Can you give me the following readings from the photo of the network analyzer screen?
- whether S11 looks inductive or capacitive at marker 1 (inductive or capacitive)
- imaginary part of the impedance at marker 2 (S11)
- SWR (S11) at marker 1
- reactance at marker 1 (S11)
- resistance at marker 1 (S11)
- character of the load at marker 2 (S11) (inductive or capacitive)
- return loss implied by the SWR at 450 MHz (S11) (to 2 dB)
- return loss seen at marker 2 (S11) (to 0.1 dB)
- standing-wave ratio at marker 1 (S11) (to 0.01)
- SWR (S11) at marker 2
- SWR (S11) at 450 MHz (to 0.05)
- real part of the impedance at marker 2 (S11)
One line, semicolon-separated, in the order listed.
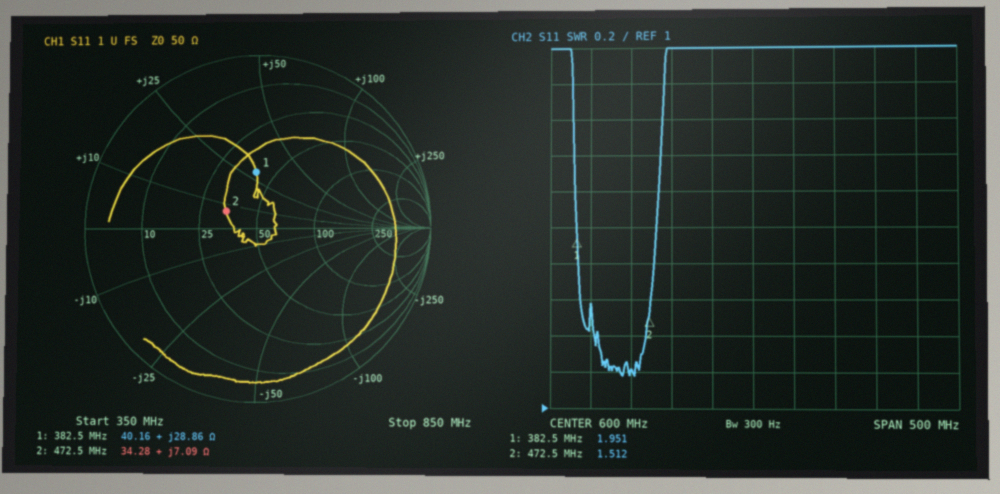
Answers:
inductive; +7.09 Ω; 1.951; +28.86 Ω; 40.16 Ω; inductive; 20 dB; 13.8 dB; 1.95; 1.512; 1.20; 34.28 Ω
